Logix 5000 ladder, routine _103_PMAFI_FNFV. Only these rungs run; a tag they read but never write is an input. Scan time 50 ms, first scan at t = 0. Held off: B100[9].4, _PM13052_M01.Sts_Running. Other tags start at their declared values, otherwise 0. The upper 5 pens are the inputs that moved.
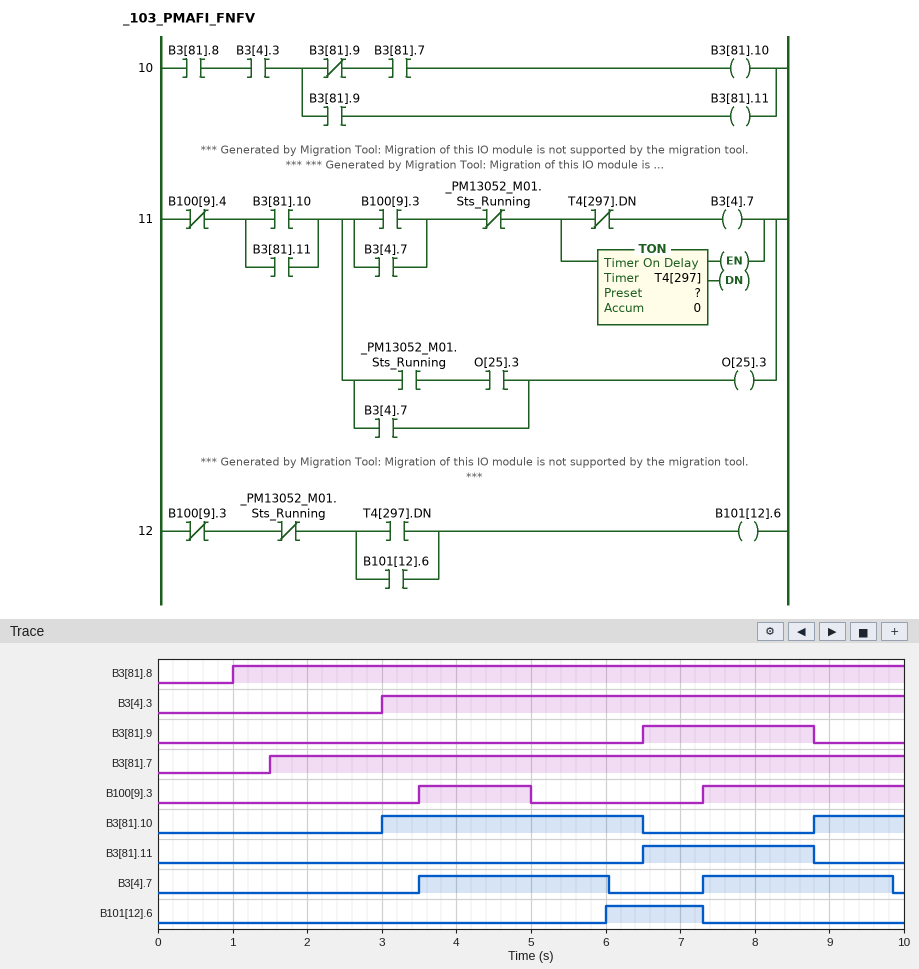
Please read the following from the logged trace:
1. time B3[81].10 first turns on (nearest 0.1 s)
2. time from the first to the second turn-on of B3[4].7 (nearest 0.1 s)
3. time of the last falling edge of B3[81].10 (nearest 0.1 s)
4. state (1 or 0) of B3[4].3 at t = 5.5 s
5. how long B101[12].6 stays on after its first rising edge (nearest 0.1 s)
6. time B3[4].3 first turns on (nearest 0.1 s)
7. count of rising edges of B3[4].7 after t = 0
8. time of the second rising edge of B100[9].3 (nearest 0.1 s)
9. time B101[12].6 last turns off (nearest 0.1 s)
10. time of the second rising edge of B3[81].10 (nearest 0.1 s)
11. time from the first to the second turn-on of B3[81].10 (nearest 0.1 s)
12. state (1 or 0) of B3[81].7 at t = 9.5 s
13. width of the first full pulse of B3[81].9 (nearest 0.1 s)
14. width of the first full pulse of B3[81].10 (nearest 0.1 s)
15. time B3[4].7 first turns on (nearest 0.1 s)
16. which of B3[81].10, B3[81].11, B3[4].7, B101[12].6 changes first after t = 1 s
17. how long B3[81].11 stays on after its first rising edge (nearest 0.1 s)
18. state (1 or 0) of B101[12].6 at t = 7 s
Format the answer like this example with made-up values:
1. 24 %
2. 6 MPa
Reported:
1. 3.0 s
2. 3.8 s
3. 6.5 s
4. 1
5. 1.3 s
6. 3.0 s
7. 2
8. 7.3 s
9. 7.3 s
10. 8.8 s
11. 5.8 s
12. 1
13. 2.3 s
14. 3.5 s
15. 3.5 s
16. B3[81].10
17. 2.3 s
18. 1
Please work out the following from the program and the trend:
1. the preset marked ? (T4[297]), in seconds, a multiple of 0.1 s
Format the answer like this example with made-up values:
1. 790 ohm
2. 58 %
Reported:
1. 2.5 s
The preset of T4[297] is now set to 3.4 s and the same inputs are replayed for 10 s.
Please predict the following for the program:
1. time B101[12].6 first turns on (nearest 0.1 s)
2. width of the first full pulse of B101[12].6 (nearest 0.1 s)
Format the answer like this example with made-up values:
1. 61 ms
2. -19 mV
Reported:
1. 6.9 s
2. 0.4 s
